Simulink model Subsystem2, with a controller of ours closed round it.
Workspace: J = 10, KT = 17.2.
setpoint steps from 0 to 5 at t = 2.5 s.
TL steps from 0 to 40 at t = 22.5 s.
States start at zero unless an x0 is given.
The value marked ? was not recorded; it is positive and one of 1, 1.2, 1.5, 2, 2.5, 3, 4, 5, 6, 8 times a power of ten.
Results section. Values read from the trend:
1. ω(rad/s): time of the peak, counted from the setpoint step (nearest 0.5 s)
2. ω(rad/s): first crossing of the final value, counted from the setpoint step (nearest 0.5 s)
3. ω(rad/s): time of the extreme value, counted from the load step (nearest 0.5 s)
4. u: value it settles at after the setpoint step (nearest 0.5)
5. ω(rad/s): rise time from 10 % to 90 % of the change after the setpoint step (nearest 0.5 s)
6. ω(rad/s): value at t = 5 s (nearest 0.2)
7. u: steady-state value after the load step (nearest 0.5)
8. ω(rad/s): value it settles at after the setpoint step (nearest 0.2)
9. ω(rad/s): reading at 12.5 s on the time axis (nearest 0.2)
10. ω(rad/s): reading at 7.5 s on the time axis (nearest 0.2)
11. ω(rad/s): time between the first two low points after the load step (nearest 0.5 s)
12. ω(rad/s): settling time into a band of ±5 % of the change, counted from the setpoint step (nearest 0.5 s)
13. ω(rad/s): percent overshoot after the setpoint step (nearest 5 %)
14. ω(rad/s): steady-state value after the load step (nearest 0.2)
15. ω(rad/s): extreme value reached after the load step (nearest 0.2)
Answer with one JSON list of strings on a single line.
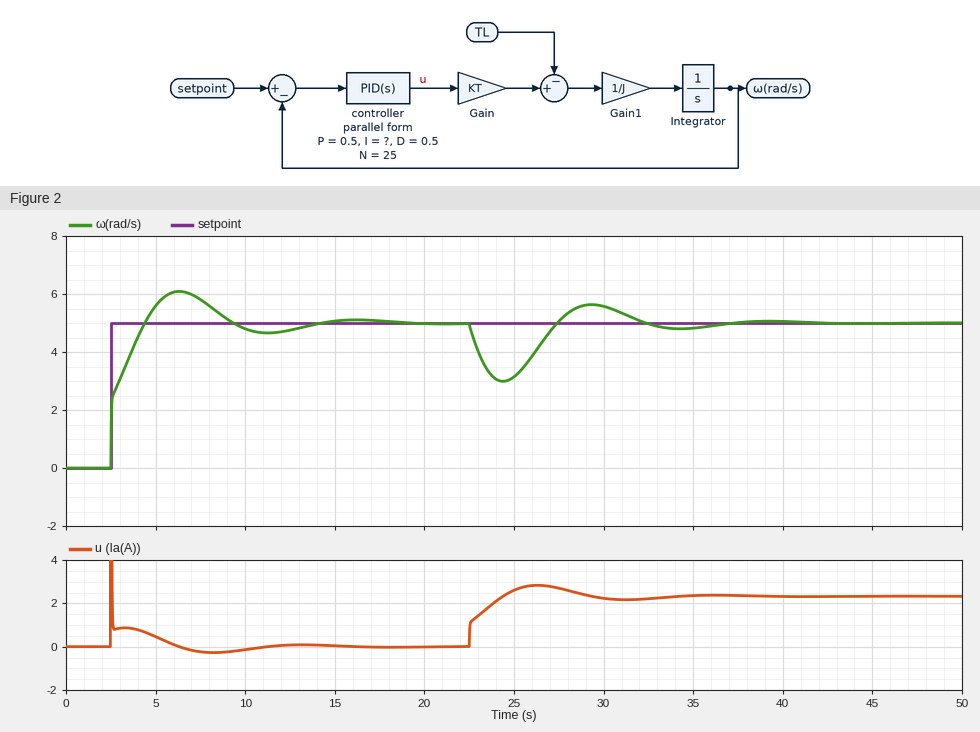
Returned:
["4.0 s", "2.0 s", "2.0 s", "0.0", "1.5 s", "5.6", "2.5", "5.0", "4.8", "5.8", "10.0 s", "10.0 s", "20 %", "5.0", "3.0"]
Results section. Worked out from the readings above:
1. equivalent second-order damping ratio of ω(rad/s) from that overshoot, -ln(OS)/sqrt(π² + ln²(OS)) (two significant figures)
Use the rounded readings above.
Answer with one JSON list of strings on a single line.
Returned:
["0.46"]
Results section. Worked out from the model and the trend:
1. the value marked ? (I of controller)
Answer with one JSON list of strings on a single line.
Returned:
["0.5"]
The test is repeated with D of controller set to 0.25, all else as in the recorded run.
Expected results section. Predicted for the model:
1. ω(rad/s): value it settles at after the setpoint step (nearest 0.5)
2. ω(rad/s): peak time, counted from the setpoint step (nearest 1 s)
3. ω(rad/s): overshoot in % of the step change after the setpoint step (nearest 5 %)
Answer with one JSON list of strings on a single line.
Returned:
["5.0", "3 s", "25 %"]
